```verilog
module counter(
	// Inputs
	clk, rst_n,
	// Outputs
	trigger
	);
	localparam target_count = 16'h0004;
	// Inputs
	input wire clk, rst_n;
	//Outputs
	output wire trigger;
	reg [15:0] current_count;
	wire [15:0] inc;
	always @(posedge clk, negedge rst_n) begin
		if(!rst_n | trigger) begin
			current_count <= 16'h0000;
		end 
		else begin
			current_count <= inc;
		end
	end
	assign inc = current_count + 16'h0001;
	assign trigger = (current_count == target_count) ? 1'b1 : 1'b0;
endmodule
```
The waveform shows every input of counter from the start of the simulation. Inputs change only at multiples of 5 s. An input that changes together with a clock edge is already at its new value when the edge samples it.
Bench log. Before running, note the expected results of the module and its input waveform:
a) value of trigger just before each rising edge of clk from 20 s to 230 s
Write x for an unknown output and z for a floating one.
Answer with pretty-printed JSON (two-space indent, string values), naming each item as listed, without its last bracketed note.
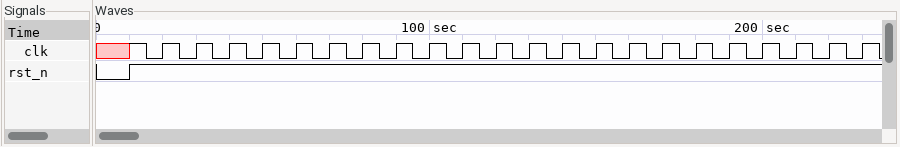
{
  "value of trigger just before each rising edge of clk from 20 s to 230 s": "0 0 0 1 0 0 0 0 1 0 0 0 0 1 0 0 0 0 1 0 0 0"
}
